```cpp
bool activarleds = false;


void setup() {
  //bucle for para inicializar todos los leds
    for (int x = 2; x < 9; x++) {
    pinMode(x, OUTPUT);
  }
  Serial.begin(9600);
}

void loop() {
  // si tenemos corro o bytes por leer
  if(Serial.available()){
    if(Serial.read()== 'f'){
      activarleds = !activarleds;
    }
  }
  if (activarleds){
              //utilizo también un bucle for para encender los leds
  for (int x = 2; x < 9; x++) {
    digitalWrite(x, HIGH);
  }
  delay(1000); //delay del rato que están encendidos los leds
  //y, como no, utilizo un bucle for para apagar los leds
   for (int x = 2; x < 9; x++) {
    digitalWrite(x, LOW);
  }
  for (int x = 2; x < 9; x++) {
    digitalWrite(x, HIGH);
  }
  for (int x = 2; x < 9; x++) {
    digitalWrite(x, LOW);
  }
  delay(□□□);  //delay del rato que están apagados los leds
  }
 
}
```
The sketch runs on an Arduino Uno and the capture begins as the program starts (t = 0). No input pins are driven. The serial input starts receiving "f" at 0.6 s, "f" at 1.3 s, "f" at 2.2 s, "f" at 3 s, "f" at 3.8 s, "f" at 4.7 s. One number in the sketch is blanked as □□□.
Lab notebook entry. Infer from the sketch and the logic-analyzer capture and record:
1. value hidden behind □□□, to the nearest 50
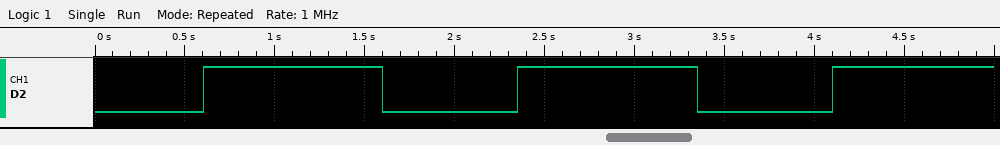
750
